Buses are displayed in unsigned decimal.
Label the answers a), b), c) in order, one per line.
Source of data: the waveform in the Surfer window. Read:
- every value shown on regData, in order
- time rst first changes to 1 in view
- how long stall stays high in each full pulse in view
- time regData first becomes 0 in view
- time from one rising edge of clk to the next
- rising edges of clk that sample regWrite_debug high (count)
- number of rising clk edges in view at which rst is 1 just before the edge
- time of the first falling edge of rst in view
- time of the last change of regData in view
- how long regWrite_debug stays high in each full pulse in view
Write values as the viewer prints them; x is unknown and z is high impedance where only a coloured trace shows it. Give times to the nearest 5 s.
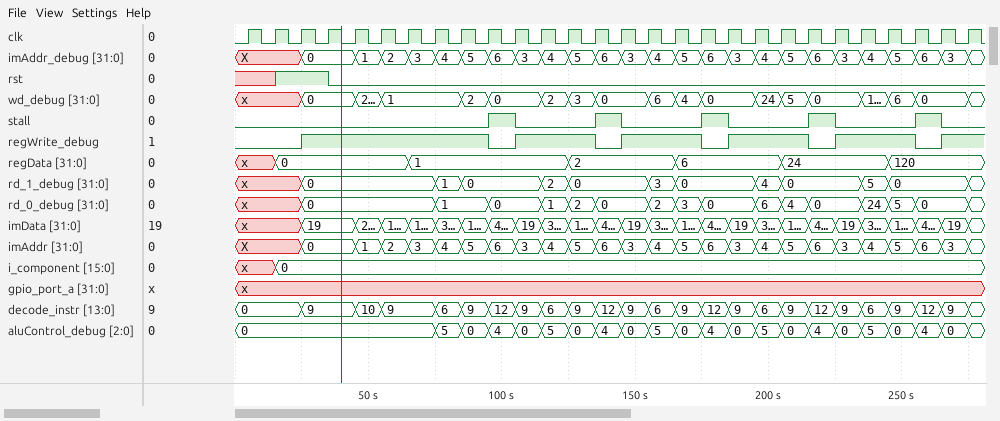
a) x, 0, 1, 2, 6, 24, 120
b) 15 s
c) 10 s, 10 s, 10 s, 10 s, 10 s
d) 15 s
e) 10 s
f) 20
g) 2
h) 35 s
i) 245 s
j) 70 s, 30 s, 30 s, 30 s, 30 s
